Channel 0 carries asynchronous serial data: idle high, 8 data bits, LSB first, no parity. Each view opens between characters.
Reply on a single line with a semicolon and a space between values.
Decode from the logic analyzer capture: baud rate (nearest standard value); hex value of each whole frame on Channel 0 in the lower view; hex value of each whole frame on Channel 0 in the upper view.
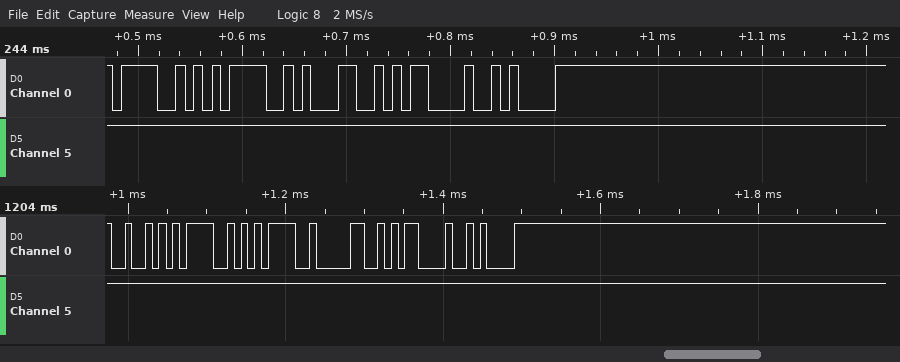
115200 baud; 52, 4F, 3D, 30, 0D, 0A; 4F, 3D, 31, 0D, 0A
